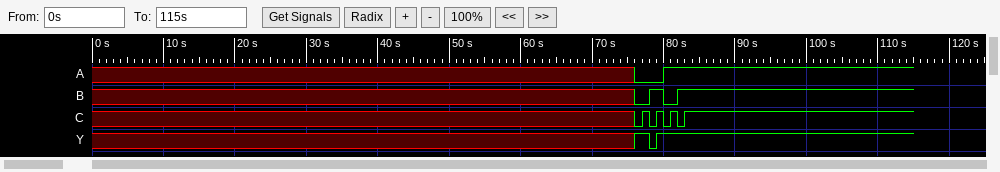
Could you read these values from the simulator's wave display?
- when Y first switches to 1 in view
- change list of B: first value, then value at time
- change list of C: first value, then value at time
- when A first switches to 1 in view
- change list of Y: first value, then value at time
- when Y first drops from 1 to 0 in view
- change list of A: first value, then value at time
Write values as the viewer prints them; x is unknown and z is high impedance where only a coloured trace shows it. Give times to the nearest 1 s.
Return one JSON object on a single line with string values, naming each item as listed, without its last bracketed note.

{"when Y first switches to 1 in view": "76 s", "change list of B: first value, then value at time": "x, 0 at 76 s, 1 at 78 s, 0 at 80 s, 1 at 82 s", "change list of C: first value, then value at time": "x, 0 at 76 s, 1 at 77 s, 0 at 78 s, 1 at 79 s, 0 at 80 s, 1 at 81 s, 0 at 82 s, 1 at 83 s", "when A first switches to 1 in view": "80 s", "change list of Y: first value, then value at time": "x, 1 at 76 s, 0 at 78 s, 1 at 79 s", "when Y first drops from 1 to 0 in view": "78 s", "change list of A: first value, then value at time": "x, 0 at 76 s, 1 at 80 s"}
